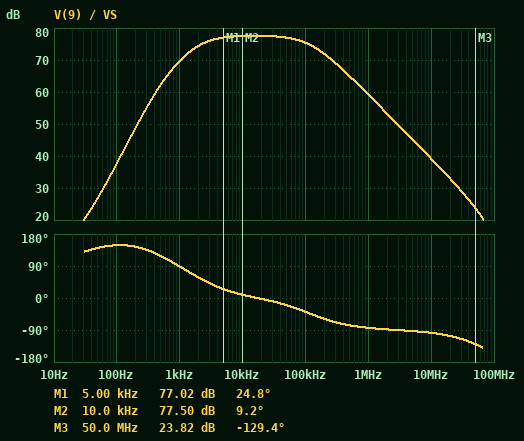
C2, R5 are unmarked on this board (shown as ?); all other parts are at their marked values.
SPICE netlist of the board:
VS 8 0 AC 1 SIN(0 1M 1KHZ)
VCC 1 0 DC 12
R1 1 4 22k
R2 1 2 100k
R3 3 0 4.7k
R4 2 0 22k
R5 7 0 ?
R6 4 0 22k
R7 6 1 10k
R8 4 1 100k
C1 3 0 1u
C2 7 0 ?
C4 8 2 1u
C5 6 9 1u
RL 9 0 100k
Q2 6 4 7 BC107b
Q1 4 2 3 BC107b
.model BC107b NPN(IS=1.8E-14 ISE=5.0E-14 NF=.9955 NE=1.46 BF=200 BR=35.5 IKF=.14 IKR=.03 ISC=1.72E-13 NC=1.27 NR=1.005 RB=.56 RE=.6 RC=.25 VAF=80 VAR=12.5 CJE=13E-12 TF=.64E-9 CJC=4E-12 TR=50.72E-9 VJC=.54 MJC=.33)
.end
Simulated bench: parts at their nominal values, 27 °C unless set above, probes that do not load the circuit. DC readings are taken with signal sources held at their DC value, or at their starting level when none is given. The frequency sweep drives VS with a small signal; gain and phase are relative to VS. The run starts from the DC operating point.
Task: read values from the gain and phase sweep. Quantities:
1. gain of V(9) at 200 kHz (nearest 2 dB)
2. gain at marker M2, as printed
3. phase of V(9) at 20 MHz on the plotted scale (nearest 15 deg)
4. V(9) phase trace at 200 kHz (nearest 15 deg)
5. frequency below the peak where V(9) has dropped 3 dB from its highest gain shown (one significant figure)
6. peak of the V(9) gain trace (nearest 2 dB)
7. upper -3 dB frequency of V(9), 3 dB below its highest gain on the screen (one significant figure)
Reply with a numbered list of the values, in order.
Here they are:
1. 72 dB
2. 77.50 dB
3. -105 deg
4. -60 deg
5. 2 kHz
6. 78 dB
7. 100 kHz
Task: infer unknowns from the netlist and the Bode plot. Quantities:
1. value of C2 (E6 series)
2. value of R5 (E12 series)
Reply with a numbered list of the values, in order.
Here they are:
1. 2.2 µF
2. 8.2 kΩ
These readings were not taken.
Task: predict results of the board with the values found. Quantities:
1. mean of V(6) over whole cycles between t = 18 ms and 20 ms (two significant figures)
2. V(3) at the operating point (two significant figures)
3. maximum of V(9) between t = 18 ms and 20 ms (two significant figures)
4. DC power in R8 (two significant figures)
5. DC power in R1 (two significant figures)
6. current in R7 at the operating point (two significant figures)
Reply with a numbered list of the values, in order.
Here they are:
1. 8.6 V
2. 1.5 V
3. 2.4 V
4. 740 µW
5. 3.4 mW
6. 340 µA
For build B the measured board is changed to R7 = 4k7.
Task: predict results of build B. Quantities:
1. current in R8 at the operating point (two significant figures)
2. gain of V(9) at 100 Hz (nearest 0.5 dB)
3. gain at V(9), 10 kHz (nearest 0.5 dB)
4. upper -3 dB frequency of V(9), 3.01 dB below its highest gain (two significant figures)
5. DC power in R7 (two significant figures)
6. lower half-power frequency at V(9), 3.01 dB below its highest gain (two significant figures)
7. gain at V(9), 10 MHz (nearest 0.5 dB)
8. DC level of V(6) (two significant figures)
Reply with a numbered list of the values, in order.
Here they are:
1. 86 µA
2. 31.5 dB
3. 71.5 dB
4. 230 kHz
5. 540 µW
6. 2.1 kHz
7. 38.5 dB
8. 10 V
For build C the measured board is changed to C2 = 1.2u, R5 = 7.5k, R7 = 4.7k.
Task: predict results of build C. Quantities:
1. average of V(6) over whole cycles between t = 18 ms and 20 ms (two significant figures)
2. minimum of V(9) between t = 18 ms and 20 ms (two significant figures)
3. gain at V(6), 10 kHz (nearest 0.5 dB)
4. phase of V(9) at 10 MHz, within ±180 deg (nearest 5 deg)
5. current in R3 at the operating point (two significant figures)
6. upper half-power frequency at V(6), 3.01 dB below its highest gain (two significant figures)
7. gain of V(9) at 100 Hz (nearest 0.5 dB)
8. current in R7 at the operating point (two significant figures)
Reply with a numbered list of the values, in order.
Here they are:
1. 10 V
2. -1.3 V
3. 72.0 dB
4. -95 deg
5. 320 µA
6. 220 kHz
7. 26.5 dB
8. 370 µA
